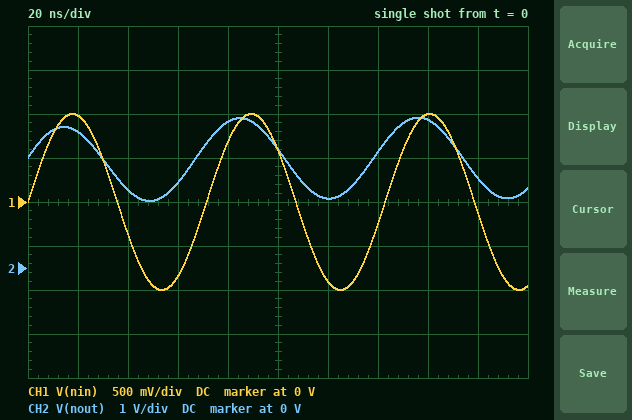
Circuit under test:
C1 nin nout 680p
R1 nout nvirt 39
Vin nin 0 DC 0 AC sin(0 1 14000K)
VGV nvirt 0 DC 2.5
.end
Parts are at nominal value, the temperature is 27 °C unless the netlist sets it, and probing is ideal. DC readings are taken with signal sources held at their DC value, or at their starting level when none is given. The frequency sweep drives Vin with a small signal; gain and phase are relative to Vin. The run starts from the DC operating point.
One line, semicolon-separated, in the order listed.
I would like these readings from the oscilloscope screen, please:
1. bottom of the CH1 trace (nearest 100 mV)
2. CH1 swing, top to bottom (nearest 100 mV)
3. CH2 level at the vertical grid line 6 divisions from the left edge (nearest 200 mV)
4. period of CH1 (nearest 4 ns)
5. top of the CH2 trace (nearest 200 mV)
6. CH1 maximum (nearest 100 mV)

-1.0 V; 2.0 V; 1.6 V; 72 ns; 3.4 V; 1.0 V
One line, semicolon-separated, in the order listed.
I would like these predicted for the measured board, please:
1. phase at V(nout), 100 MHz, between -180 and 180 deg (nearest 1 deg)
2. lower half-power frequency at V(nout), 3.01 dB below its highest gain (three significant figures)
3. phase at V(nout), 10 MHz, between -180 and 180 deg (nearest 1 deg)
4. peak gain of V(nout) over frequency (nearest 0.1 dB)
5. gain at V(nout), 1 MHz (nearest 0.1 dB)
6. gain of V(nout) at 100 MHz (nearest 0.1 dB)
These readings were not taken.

3 deg; 6.00 MHz; 31 deg; 0 dB; -15.7 dB; 0 dB
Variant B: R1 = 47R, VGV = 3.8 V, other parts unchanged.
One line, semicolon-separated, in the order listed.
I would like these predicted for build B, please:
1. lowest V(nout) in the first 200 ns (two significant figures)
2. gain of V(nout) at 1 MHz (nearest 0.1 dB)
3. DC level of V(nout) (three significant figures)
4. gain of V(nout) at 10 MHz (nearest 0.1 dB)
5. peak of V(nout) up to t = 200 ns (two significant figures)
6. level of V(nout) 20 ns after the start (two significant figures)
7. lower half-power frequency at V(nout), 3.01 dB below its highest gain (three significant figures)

2.8 V; -14.1 dB; 3.80 V; -1.0 dB; 4.7 V; 4.4 V; 4.98 MHz
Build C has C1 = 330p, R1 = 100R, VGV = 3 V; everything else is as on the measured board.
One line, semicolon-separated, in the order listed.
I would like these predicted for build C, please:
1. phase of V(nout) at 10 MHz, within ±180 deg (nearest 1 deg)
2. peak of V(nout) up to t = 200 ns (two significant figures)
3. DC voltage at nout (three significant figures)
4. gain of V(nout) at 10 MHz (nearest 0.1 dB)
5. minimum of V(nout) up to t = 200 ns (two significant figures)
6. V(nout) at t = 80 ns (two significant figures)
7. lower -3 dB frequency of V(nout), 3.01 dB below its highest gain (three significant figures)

26 deg; 3.9 V; 3.00 V; -0.9 dB; 2.0 V; 3.8 V; 4.82 MHz
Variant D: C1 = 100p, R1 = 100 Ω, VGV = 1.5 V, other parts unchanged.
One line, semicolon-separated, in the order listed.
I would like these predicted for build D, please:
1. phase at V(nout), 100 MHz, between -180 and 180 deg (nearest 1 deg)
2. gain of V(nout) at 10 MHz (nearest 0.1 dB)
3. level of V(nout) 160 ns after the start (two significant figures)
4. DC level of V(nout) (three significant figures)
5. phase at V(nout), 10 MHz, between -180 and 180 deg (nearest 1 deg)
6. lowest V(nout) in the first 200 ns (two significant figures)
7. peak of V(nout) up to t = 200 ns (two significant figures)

9 deg; -5.5 dB; 2.0 V; 1.50 V; 58 deg; 830 mV; 2.2 V
